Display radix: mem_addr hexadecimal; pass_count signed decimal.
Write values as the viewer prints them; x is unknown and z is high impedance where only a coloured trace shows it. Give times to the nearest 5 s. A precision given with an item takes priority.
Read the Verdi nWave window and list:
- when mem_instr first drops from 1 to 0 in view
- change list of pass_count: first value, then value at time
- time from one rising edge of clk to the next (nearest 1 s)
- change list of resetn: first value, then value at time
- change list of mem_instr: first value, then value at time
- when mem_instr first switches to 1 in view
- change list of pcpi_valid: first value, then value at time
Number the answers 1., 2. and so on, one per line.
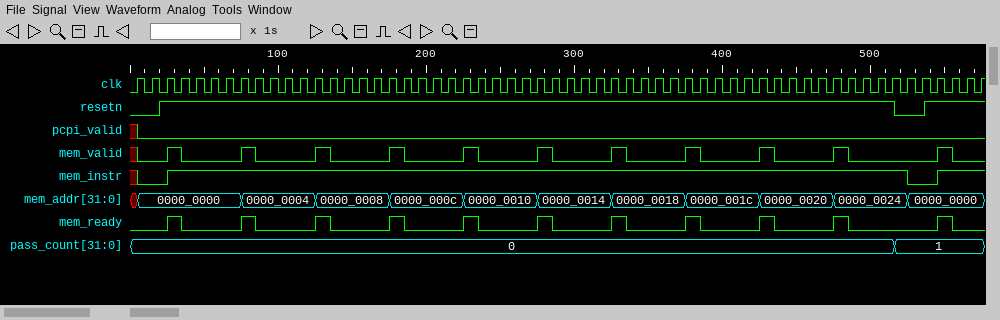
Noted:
1. 525 s
2. 0, 1 at 515 s
3. 10 s
4. 0, 1 at 20 s, 0 at 515 s, 1 at 535 s
5. x, 0 at 5 s, 1 at 25 s, 0 at 525 s, 1 at 545 s
6. 25 s
7. x, 0 at 5 s
